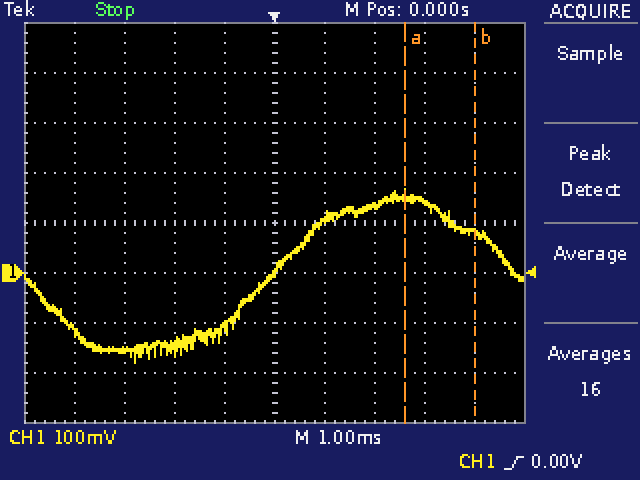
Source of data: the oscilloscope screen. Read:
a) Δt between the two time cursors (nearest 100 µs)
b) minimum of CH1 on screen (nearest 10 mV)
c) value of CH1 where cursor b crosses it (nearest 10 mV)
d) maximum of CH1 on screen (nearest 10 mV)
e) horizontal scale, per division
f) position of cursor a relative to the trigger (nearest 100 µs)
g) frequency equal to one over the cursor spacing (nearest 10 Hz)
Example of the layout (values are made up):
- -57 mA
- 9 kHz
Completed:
- 1.4 ms
- -180 mV
- 80 mV
- 170 mV
- 1 ms
- +2.6 ms
- 710 Hz
